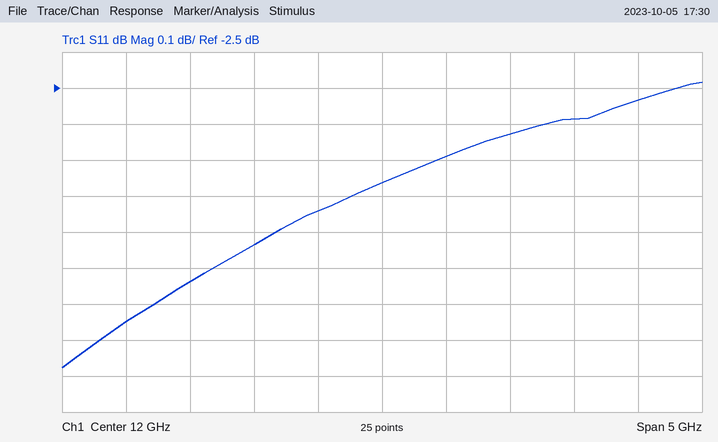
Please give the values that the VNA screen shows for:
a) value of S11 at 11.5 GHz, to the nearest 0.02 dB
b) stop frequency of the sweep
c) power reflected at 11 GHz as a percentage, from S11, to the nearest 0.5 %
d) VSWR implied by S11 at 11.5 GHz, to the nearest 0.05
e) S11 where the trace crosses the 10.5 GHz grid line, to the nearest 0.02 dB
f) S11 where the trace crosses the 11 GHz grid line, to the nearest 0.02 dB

-2.84 dB
14.5 GHz
51.0 %
6.15
-3.04 dB
-2.94 dB
